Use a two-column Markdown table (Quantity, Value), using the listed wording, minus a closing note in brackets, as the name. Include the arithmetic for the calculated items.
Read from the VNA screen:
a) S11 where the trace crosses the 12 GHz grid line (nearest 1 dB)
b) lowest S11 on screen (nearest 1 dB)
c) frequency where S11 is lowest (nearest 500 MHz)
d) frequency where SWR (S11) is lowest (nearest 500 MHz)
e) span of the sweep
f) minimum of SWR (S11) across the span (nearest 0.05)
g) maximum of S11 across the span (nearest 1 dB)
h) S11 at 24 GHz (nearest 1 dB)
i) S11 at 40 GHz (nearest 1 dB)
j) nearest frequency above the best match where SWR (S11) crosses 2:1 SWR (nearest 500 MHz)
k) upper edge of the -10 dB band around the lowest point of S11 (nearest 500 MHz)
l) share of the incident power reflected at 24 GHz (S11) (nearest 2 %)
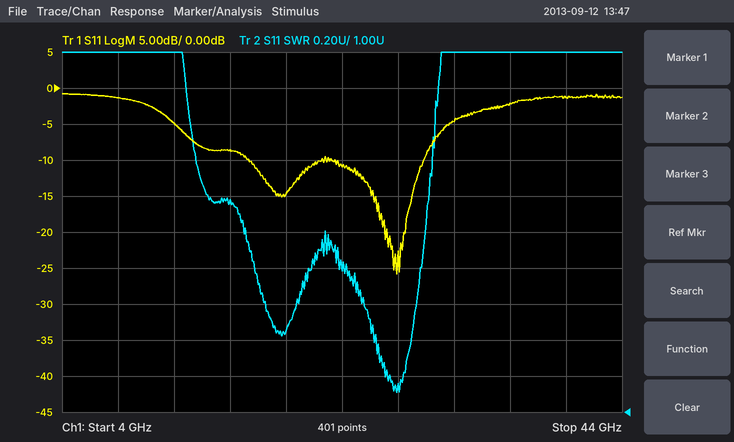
| Quantity | Value |
|---|---|
| S11 where the trace crosses the 12 GHz grid line | -5 dB |
| lowest S11 on screen | -26 dB |
| frequency where S11 is lowest | 28.0 GHz |
| frequency where SWR (S11) is lowest | 28.0 GHz |
| span of the sweep | 40 GHz |
| minimum of SWR (S11) across the span | 1.10 |
| maximum of S11 across the span | -1 dB |
| S11 at 24 GHz | -11 dB |
| S11 at 40 GHz | -1 dB |
| nearest frequency above the best match where SWR (S11) crosses 2:1 SWR | 30.0 GHz |
| upper edge of the -10 dB band around the lowest point of S11 | 30.0 GHz |
| share of the incident power reflected at 24 GHz (S11) | 10^(-11/10) ≈ 8 % |
